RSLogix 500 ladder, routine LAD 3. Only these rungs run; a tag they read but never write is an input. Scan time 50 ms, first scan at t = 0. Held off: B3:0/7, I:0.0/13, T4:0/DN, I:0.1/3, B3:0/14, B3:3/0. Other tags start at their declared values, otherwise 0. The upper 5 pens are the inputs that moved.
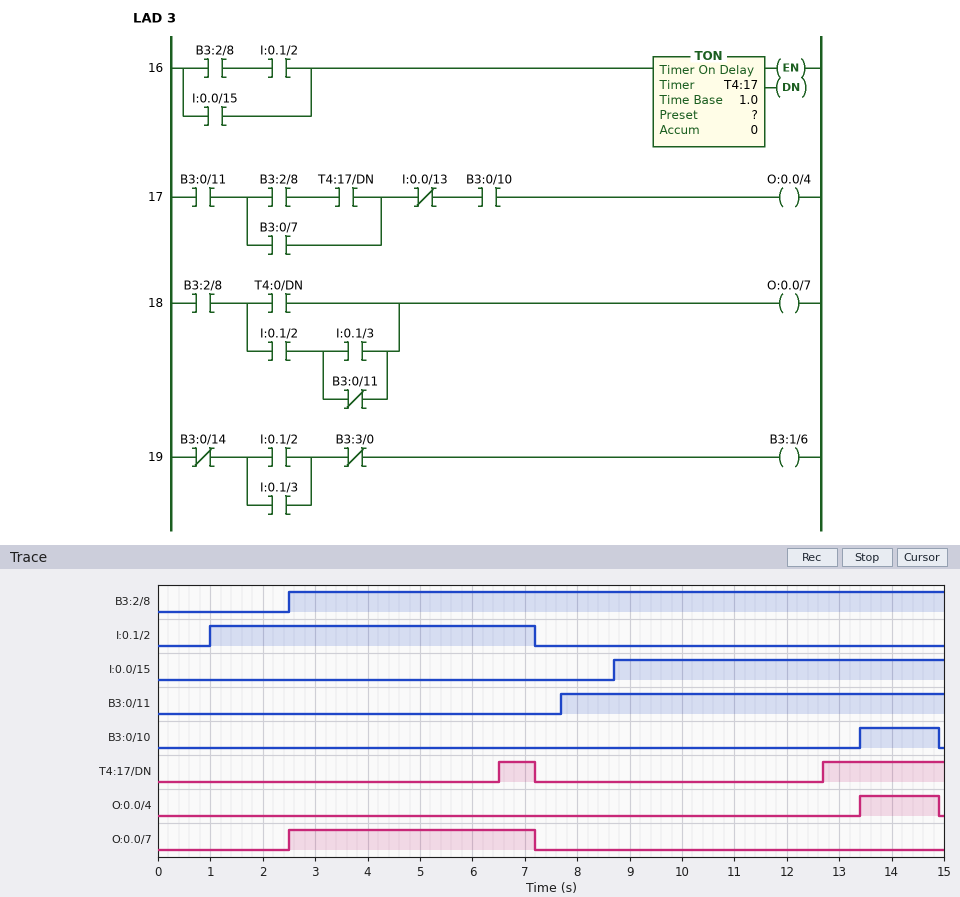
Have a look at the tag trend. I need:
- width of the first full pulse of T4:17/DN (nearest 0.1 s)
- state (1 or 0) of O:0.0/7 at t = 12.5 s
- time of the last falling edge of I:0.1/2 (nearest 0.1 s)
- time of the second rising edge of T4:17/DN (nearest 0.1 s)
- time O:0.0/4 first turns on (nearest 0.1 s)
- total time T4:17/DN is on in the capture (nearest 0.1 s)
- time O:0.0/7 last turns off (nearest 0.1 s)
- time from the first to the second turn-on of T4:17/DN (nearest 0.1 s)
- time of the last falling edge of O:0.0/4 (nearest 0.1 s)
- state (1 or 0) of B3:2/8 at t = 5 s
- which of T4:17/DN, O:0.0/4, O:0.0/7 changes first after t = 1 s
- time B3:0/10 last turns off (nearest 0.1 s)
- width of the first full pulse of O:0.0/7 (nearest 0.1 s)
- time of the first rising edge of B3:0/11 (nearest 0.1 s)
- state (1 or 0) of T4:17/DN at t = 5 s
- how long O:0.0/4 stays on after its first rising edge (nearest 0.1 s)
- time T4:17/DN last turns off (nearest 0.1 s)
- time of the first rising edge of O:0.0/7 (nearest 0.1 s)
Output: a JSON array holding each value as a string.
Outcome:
["0.7 s", "0", "7.2 s", "12.7 s", "13.4 s", "3.0 s", "7.2 s", "6.2 s", "14.9 s", "1", "O:0.0/7", "14.9 s", "4.7 s", "7.7 s", "0", "1.5 s", "7.2 s", "2.5 s"]
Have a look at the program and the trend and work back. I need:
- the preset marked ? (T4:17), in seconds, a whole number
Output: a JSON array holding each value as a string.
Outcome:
["4 s"]
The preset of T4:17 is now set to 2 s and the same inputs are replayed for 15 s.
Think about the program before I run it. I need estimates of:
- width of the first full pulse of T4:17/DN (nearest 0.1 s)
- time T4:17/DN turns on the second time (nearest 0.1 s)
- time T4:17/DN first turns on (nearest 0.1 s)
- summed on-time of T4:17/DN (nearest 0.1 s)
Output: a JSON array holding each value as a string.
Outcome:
["2.7 s", "10.7 s", "4.5 s", "7.0 s"]
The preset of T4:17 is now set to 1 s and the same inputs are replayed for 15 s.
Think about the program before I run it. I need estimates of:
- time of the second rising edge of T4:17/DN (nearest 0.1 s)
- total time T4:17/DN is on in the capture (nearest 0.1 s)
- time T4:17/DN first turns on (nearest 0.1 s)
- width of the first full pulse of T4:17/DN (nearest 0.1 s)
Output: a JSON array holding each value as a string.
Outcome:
["9.7 s", "9.0 s", "3.5 s", "3.7 s"]
